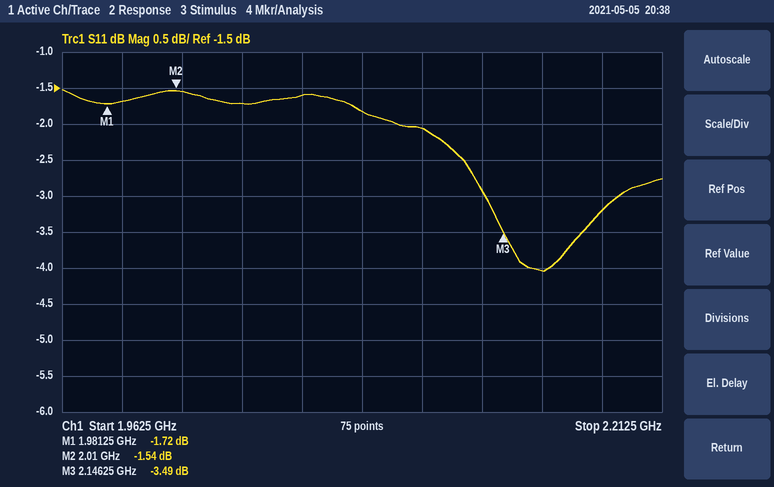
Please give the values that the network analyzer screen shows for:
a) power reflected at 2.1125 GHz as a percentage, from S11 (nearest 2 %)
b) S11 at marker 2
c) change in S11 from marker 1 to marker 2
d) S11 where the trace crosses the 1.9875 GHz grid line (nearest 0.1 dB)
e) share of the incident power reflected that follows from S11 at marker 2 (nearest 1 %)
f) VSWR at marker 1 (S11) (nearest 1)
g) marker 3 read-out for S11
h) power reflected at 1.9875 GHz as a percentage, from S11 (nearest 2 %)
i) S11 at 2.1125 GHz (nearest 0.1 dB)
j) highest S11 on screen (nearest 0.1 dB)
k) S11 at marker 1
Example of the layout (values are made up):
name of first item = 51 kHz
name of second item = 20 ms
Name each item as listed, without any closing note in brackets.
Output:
power reflected at 2.1125 GHz as a percentage, from S11 = 62 %
S11 at marker 2 = -1.54 dB
change in S11 from marker 1 to marker 2 = 0.18 dB
S11 where the trace crosses the 1.9875 GHz grid line = -1.7 dB
share of the incident power reflected that follows from S11 at marker 2 = 70 %
VSWR at marker 1 (S11) = 10
marker 3 read-out for S11 = -3.49 dB
power reflected at 1.9875 GHz as a percentage, from S11 = 68 %
S11 at 2.1125 GHz = -2.1 dB
highest S11 on screen = -1.5 dB
S11 at marker 1 = -1.72 dB
